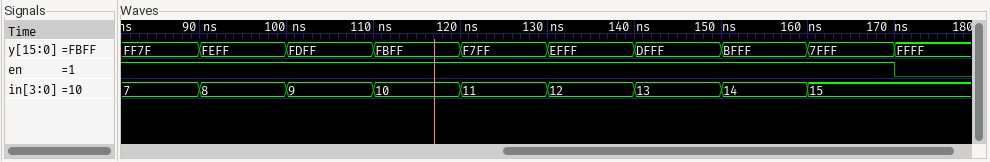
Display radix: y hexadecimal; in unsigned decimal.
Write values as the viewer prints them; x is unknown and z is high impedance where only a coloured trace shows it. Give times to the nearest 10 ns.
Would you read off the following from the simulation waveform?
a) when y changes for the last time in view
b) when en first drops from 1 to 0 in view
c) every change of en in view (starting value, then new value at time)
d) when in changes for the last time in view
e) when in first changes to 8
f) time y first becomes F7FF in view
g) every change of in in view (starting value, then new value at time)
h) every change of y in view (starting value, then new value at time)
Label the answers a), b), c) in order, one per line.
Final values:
a) 170 ns
b) 170 ns
c) 1, 0 at 170 ns
d) 160 ns
e) 90 ns
f) 120 ns
g) 7, 8 at 90 ns, 9 at 100 ns, 10 at 110 ns, 11 at 120 ns, 12 at 130 ns, 13 at 140 ns, 14 at 150 ns, 15 at 160 ns
h) FF7F, FEFF at 90 ns, FDFF at 100 ns, FBFF at 110 ns, F7FF at 120 ns, EFFF at 130 ns, DFFF at 140 ns, BFFF at 150 ns, 7FFF at 160 ns, FFFF at 170 ns
